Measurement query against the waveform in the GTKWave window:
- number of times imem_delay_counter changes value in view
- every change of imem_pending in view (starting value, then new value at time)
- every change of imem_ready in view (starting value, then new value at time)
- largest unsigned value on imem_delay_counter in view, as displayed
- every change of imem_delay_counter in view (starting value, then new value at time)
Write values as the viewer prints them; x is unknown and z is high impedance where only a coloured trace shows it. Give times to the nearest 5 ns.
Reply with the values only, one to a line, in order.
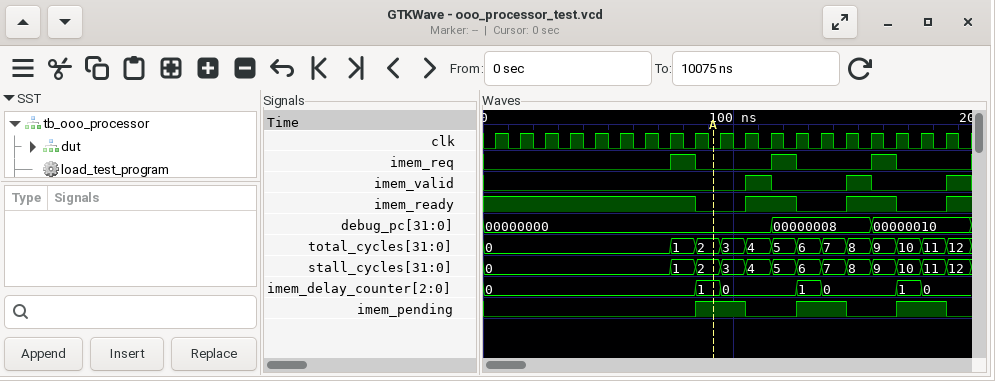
6
0, 1 at 85 ns, 0 at 105 ns, 1 at 125 ns, 0 at 145 ns, 1 at 165 ns, 0 at 185 ns
1, 0 at 85 ns, 1 at 105 ns, 0 at 125 ns, 1 at 145 ns, 0 at 165 ns, 1 at 185 ns
1
0, 1 at 85 ns, 0 at 95 ns, 1 at 125 ns, 0 at 135 ns, 1 at 165 ns, 0 at 175 ns
